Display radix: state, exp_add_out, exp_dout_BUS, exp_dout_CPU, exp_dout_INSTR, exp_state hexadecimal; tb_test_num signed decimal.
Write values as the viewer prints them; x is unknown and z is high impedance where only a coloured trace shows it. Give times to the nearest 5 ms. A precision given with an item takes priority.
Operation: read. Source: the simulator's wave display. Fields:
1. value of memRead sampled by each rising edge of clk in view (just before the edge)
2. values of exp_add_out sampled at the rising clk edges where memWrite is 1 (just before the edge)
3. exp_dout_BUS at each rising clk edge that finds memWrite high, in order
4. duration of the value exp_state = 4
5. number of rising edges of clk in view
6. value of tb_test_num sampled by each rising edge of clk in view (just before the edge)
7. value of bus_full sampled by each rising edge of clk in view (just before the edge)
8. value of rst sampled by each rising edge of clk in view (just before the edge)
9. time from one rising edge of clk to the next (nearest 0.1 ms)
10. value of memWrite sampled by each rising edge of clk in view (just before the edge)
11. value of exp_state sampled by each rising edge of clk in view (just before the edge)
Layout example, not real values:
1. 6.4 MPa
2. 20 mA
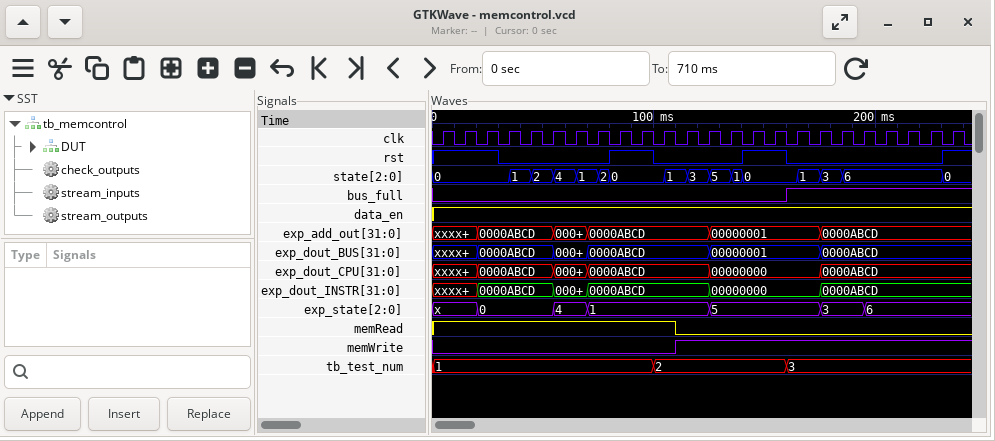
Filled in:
1. 1 1 1 1 1 1 1 1 1 1 1 0 0 0 0 0 0 0 0 0 0 0 0 0
2. 0000ABCD, 0000ABCD, 00000001, 00000001, 00000001, 00000001, 00000001, 0000ABCD, 0000ABCD, 0000ABCD, 0000ABCD, 0000ABCD, 0000ABCD
3. 0000ABCD, 0000ABCD, 00000001, 00000001, 00000001, 00000001, 00000001, 0000ABCD, 0000ABCD, 0000ABCD, 0000ABCD, 0000ABCD, 0000ABCD
4. 15 ms
5. 24
6. 1, 1, 1, 1, 1, 1, 1, 1, 1, 1, 2, 2, 2, 2, 2, 2, 3, 3, 3, 3, 3, 3, 3, 3
7. 0 0 0 0 0 0 0 0 0 0 0 0 0 0 0 0 1 1 1 1 1 1 1 1
8. 1 1 1 0 0 0 0 0 1 1 0 0 0 0 1 1 0 0 0 0 0 0 0 1
9. 10 ms
10. 0 0 0 0 0 0 0 0 0 0 0 1 1 1 1 1 1 1 1 1 1 1 1 1
11. x, x, 0, 0, 0, 0, 4, 1, 1, 1, 1, 1, 1, 5, 5, 5, 5, 5, 3, 3, 6, 6, 6, 6
